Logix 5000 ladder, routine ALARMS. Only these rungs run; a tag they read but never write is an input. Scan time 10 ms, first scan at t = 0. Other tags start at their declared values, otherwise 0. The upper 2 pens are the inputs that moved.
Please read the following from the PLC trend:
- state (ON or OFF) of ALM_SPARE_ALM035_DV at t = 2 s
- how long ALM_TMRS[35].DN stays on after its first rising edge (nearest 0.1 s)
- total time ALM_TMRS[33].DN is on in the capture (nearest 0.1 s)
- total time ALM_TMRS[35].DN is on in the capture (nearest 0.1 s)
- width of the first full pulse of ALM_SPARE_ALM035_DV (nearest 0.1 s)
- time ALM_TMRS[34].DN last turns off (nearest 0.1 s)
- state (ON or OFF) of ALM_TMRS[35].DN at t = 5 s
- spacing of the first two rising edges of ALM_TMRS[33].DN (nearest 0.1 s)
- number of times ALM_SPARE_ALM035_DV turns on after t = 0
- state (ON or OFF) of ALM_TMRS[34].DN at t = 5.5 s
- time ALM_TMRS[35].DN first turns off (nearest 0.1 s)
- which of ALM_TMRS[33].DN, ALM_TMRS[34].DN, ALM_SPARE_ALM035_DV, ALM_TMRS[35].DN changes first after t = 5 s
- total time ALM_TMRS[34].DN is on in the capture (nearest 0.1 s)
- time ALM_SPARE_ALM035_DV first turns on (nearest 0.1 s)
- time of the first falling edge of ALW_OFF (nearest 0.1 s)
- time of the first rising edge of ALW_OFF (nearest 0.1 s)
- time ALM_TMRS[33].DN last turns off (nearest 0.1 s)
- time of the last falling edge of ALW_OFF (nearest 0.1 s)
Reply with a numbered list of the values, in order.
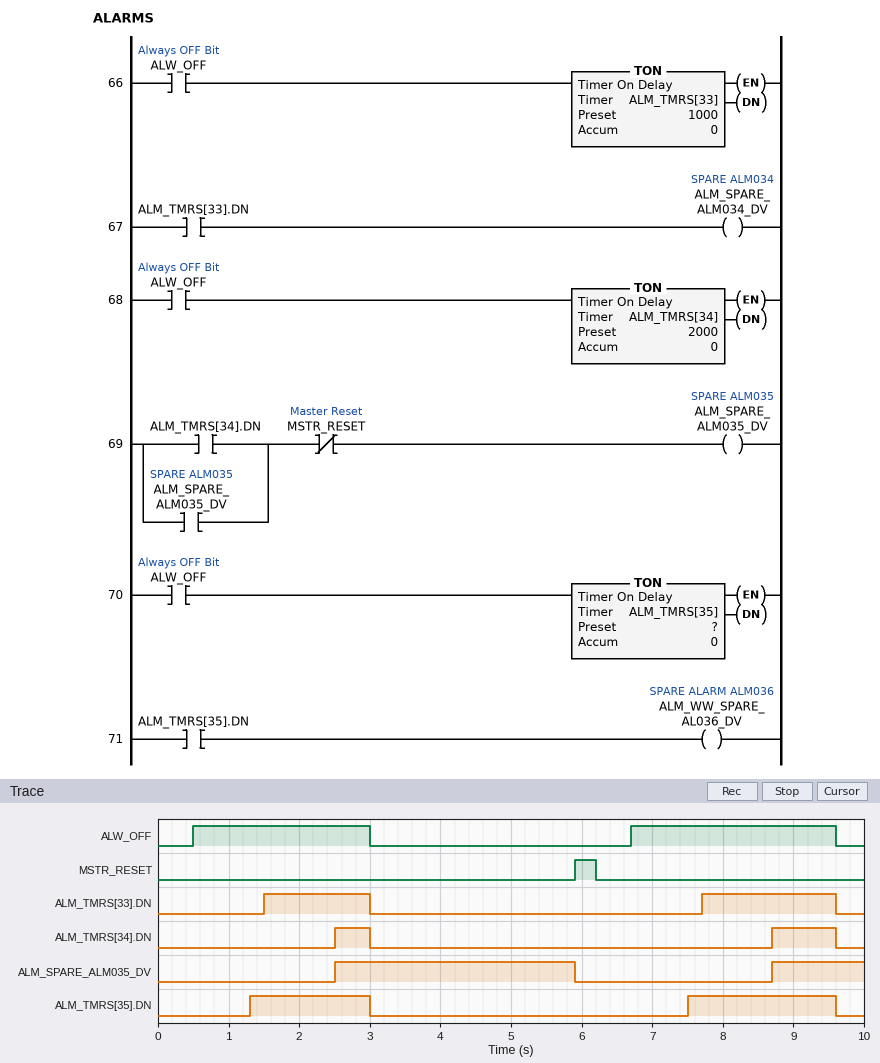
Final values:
1. OFF
2. 1.7 s
3. 3.4 s
4. 3.8 s
5. 3.4 s
6. 9.6 s
7. OFF
8. 6.2 s
9. 2
10. OFF
11. 3.0 s
12. ALM_SPARE_ALM035_DV
13. 1.4 s
14. 2.5 s
15. 3.0 s
16. 0.5 s
17. 9.6 s
18. 9.6 s
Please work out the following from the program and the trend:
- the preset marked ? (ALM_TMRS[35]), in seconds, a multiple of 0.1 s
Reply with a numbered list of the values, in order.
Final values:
1. 0.8 s
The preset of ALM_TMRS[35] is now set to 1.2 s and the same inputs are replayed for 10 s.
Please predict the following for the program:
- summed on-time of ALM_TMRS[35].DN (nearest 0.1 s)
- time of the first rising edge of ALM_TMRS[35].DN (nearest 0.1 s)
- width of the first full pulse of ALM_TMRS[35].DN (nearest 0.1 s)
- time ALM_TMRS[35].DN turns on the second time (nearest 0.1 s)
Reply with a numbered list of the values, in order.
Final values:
1. 3.0 s
2. 1.7 s
3. 1.3 s
4. 7.9 s
